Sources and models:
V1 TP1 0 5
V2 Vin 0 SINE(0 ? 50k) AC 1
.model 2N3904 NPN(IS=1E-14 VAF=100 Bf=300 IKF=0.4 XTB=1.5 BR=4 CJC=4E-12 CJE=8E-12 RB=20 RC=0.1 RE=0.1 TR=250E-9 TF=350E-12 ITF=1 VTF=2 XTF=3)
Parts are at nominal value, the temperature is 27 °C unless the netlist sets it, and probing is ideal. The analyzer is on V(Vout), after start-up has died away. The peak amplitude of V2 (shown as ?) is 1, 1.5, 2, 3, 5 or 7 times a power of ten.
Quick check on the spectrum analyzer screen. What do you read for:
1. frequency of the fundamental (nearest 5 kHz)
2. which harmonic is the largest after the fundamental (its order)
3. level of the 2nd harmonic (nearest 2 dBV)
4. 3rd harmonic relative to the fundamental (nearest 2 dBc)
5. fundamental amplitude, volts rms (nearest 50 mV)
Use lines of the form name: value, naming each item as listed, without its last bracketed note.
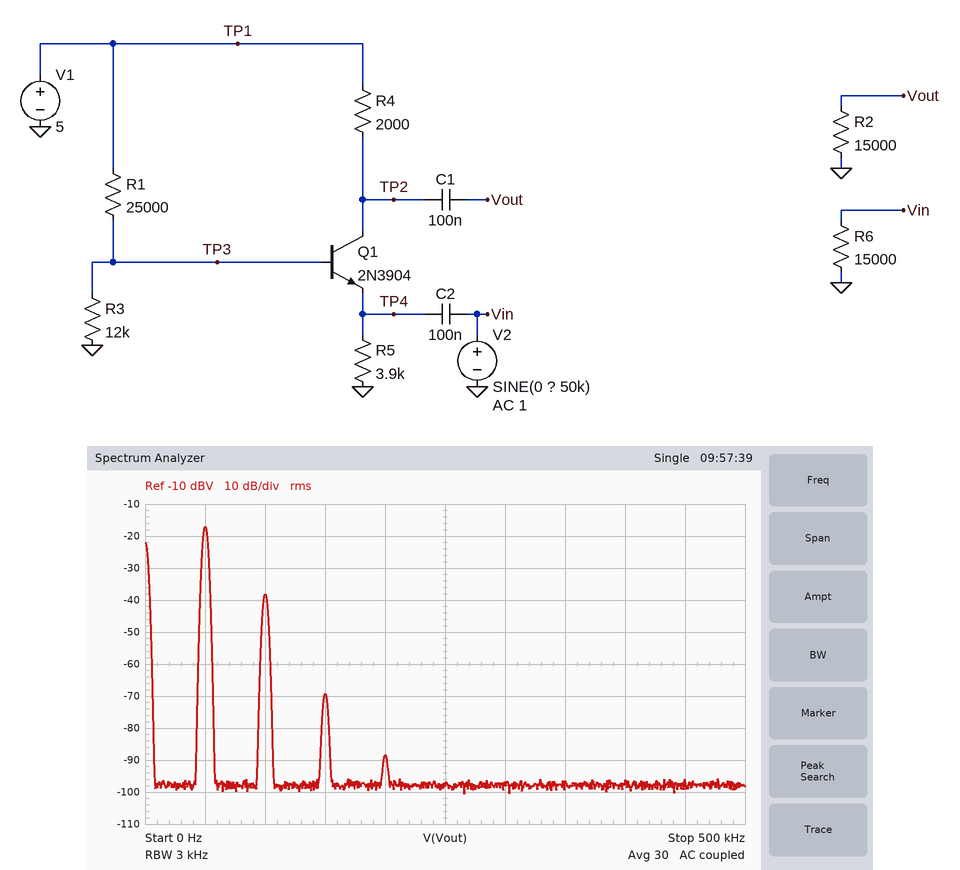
frequency of the fundamental: 50 kHz
which harmonic is the largest after the fundamental: 2
level of the 2nd harmonic: -38 dBV
3rd harmonic relative to the fundamental: -52 dBc
fundamental amplitude, volts rms: 150 mV
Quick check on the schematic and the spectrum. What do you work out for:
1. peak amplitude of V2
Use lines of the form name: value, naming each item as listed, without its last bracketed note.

peak amplitude of V2: 15 mV
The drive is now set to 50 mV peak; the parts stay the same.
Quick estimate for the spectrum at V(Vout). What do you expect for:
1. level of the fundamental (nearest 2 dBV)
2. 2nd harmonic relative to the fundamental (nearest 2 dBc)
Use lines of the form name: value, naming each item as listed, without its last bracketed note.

level of the fundamental: -8 dBV
2nd harmonic relative to the fundamental: -10 dBc
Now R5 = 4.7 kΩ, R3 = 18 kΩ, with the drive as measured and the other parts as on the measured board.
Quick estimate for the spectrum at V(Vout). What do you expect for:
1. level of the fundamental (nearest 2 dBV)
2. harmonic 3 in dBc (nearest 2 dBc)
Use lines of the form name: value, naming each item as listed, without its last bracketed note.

level of the fundamental: -16 dBV
harmonic 3 in dBc: -58 dBc
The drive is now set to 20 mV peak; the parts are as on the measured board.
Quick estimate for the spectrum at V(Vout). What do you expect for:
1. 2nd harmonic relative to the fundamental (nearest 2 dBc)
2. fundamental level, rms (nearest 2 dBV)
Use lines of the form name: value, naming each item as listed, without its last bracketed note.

2nd harmonic relative to the fundamental: -18 dBc
fundamental level, rms: -14 dBV
